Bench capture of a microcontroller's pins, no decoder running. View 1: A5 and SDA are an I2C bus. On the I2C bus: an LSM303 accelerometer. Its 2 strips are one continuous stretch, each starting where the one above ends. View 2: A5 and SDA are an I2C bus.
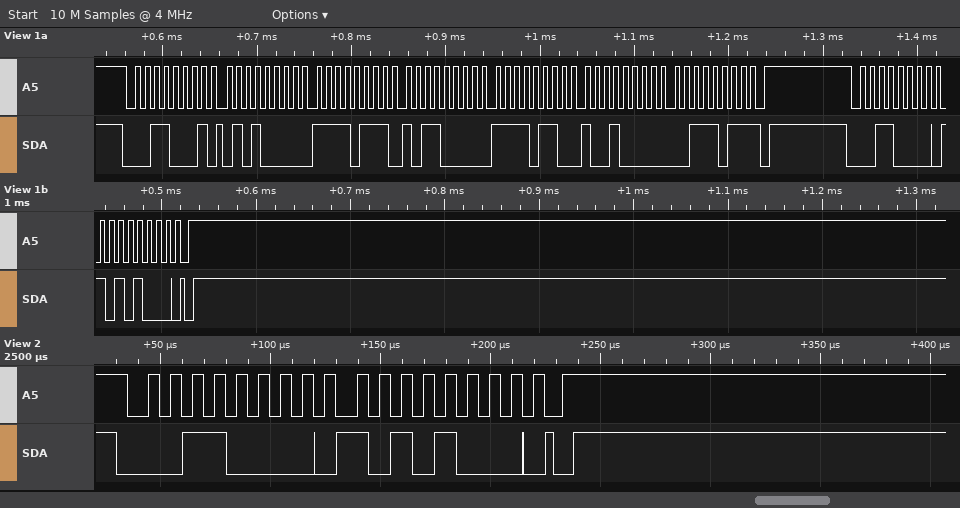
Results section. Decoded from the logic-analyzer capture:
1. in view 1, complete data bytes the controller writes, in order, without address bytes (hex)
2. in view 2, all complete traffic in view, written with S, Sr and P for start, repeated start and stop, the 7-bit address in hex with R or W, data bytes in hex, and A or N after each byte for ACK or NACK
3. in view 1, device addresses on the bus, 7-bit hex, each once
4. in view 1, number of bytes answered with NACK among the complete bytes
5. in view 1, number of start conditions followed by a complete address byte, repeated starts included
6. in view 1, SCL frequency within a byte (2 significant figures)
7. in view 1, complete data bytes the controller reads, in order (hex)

A8
S 18W A A8 A P
0x18
1
2
100 kHz
50 F7 B0 F6 90 3B
